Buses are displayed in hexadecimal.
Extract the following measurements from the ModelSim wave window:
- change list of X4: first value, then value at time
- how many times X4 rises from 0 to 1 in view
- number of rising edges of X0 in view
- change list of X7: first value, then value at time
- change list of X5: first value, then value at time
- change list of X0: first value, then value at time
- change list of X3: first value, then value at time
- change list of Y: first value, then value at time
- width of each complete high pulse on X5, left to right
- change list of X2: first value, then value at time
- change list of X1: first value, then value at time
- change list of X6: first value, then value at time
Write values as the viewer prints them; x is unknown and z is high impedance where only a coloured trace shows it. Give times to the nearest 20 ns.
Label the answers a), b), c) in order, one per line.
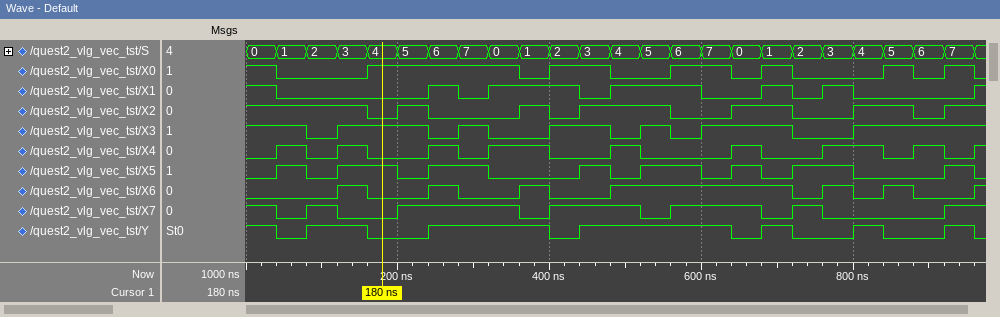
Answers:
a) 0, 1 at 40 ns, 0 at 80 ns, 1 at 120 ns, 0 at 160 ns, 1 at 240 ns, 0 at 280 ns, 1 at 320 ns, 0 at 400 ns, 1 at 480 ns, 0 at 520 ns, 1 at 640 ns, 0 at 680 ns, 1 at 760 ns, 0 at 840 ns, 1 at 880 ns, 0 at 920 ns, 1 at 960 ns
b) 9
c) 6
d) 1, 0 at 40 ns, 1 at 80 ns, 0 at 120 ns, 1 at 200 ns, 0 at 360 ns, 1 at 400 ns, 0 at 520 ns, 1 at 560 ns, 0 at 680 ns, 1 at 720 ns, 0 at 760 ns, 1 at 920 ns
e) 0, 1 at 40 ns, 0 at 80 ns, 1 at 120 ns, 0 at 200 ns, 1 at 240 ns, 0 at 320 ns, 1 at 440 ns, 0 at 480 ns, 1 at 520 ns, 0 at 600 ns, 1 at 640 ns, 0 at 680 ns, 1 at 720 ns, 0 at 800 ns, 1 at 920 ns, 0 at 960 ns
f) 1, 0 at 40 ns, 1 at 160 ns, 0 at 360 ns, 1 at 400 ns, 0 at 480 ns, 1 at 560 ns, 0 at 640 ns, 1 at 680 ns, 0 at 720 ns, 1 at 840 ns, 0 at 880 ns, 1 at 920 ns, 0 at 960 ns
g) 1, 0 at 80 ns, 1 at 120 ns, 0 at 240 ns, 1 at 280 ns, 0 at 320 ns, 1 at 400 ns, 0 at 480 ns, 1 at 520 ns, 0 at 560 ns, 1 at 600 ns, 0 at 720 ns, 1 at 800 ns
h) 1, 0 at 40 ns, 1 at 80 ns, 0 at 160 ns, 1 at 240 ns, 0 at 400 ns, 1 at 440 ns, 0 at 640 ns, 1 at 680 ns, 0 at 720 ns, 1 at 800 ns, 0 at 840 ns, 1 at 920 ns, 0 at 960 ns
i) 40 ns, 80 ns, 80 ns, 40 ns, 80 ns, 40 ns, 80 ns, 40 ns
j) 1, 0 at 160 ns, 1 at 200 ns, 0 at 240 ns, 1 at 360 ns, 0 at 400 ns, 1 at 440 ns, 0 at 560 ns, 1 at 640 ns, 0 at 720 ns, 1 at 800 ns, 0 at 880 ns, 1 at 920 ns
k) 1, 0 at 40 ns, 1 at 240 ns, 0 at 280 ns, 1 at 320 ns, 0 at 440 ns, 1 at 480 ns, 0 at 600 ns, 1 at 680 ns, 0 at 720 ns, 1 at 760 ns, 0 at 800 ns, 1 at 960 ns
l) 0, 1 at 120 ns, 0 at 160 ns, 1 at 240 ns, 0 at 280 ns, 1 at 360 ns, 0 at 400 ns, 1 at 480 ns, 0 at 720 ns, 1 at 760 ns, 0 at 800 ns, 1 at 840 ns, 0 at 880 ns, 1 at 960 ns
